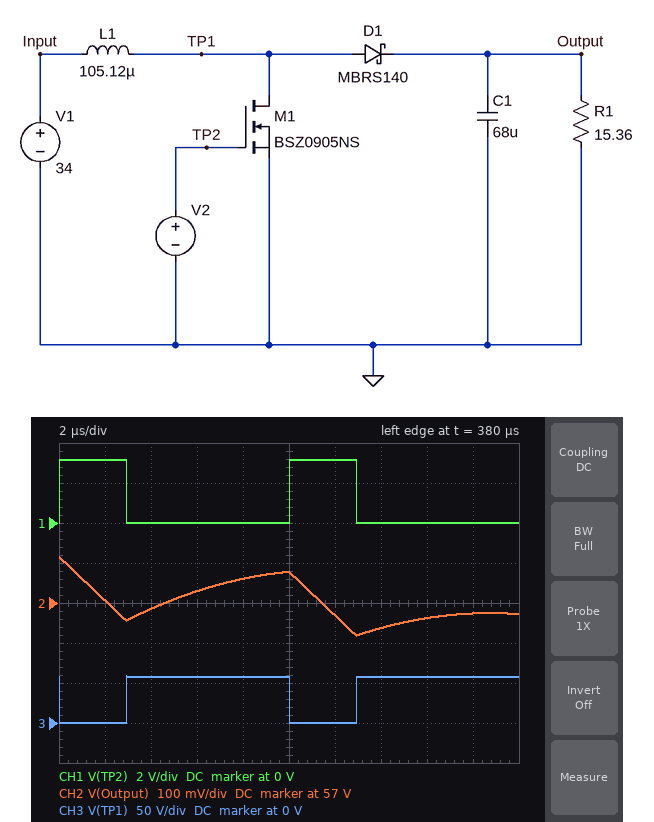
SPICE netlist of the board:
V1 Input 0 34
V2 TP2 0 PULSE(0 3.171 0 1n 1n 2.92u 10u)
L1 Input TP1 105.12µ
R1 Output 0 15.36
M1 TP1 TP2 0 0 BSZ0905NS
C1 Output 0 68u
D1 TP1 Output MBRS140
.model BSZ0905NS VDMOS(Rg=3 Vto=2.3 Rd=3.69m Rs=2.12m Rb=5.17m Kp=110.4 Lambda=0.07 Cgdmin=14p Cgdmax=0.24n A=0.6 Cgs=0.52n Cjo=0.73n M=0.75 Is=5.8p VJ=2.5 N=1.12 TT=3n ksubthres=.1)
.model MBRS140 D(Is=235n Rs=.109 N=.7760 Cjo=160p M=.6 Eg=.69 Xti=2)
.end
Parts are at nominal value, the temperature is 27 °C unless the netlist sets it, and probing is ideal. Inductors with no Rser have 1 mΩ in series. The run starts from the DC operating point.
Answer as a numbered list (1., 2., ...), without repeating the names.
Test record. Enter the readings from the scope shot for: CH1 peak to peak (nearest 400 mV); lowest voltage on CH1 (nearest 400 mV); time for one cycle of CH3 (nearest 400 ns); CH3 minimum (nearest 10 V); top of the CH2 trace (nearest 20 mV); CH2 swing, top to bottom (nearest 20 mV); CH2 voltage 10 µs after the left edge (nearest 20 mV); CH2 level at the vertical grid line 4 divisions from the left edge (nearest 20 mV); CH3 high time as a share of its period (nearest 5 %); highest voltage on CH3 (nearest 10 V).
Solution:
1. 3.2 V
2. 0 V
3. 10.0 µs
4. 0 V
5. 57.12 V
6. 200 mV
7. 57.08 V
8. 57.06 V
9. 70 %
10. 60 V
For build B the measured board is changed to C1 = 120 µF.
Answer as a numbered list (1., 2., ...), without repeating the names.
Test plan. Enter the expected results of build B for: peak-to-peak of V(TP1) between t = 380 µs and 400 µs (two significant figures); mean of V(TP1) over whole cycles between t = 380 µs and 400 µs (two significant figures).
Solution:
1. 56 V
2. 40 V
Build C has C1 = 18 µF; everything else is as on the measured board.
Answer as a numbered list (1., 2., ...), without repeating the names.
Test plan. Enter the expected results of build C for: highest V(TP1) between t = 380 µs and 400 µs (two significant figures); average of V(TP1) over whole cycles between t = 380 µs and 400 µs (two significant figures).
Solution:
1. 42 V
2. 30 V
